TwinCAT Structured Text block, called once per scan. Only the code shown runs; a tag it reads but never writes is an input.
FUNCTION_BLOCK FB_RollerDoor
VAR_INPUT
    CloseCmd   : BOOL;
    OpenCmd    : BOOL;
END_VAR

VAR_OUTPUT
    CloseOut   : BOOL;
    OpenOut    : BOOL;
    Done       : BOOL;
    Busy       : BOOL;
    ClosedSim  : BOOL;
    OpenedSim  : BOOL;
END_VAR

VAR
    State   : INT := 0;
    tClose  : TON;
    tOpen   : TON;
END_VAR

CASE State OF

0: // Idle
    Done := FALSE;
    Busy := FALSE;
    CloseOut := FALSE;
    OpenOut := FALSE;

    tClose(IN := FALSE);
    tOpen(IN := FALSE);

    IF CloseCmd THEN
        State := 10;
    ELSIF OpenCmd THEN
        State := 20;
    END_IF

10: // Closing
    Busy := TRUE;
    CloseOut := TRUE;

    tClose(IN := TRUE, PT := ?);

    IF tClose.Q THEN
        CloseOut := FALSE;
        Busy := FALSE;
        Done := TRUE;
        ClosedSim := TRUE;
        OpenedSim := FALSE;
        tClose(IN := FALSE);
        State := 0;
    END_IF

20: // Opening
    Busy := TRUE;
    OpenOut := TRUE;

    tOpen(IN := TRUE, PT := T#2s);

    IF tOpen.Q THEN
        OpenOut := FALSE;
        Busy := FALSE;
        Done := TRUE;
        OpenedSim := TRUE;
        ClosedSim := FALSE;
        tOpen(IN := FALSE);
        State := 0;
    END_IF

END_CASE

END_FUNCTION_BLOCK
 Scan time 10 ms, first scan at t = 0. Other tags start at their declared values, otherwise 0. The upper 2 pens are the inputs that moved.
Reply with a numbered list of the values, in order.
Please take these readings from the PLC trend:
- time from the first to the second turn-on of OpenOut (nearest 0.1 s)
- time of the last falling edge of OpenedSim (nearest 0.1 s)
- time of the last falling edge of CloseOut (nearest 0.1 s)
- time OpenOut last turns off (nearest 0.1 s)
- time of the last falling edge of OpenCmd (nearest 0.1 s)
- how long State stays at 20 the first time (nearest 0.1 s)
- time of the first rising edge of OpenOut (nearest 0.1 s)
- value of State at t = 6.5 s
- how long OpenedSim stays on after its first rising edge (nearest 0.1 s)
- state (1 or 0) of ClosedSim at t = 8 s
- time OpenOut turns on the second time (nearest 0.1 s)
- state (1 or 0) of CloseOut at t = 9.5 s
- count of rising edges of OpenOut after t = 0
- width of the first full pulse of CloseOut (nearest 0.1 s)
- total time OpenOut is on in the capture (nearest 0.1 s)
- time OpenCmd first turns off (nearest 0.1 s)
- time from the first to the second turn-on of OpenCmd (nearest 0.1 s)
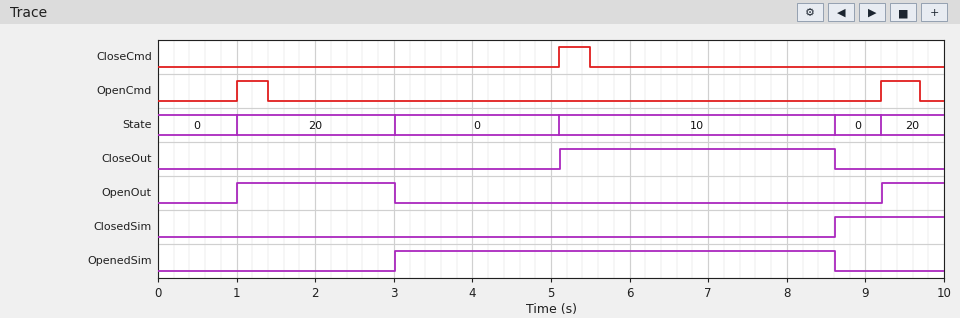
1. 8.2 s
2. 8.6 s
3. 8.6 s
4. 3.0 s
5. 9.7 s
6. 2.0 s
7. 1.0 s
8. 10
9. 5.6 s
10. 0
11. 9.2 s
12. 0
13. 2
14. 3.5 s
15. 2.8 s
16. 1.4 s
17. 8.2 s
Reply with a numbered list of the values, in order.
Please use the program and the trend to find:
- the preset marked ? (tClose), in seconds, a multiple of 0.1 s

1. 3.5 s
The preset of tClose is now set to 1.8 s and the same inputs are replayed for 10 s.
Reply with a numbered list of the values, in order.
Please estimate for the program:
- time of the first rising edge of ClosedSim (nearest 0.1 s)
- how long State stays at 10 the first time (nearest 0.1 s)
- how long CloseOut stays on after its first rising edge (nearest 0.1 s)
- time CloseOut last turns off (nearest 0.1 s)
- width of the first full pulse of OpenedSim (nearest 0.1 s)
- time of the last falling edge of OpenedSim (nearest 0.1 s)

1. 6.9 s
2. 1.8 s
3. 1.8 s
4. 6.9 s
5. 3.9 s
6. 6.9 s
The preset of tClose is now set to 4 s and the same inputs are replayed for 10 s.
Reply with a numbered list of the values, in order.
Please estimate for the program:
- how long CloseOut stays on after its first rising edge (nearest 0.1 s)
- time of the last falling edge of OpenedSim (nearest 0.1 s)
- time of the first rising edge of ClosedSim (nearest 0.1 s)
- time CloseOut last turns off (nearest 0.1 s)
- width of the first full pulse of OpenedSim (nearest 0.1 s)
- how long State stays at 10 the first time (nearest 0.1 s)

1. 4.0 s
2. 9.1 s
3. 9.1 s
4. 9.1 s
5. 6.1 s
6. 4.0 s
